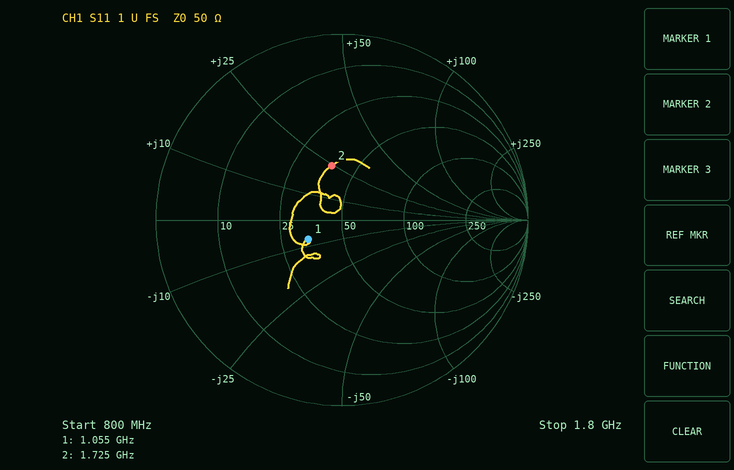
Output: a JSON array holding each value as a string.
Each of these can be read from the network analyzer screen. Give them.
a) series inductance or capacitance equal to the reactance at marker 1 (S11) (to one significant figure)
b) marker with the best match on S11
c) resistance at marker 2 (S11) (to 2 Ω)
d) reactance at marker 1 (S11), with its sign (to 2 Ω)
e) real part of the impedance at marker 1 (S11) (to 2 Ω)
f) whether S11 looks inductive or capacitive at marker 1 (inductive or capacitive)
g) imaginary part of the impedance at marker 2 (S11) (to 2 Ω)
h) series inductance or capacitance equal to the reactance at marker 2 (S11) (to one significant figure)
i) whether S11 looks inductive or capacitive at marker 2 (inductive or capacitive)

["20 pF", "marker 1", "38 Ω", "-8 Ω", "34 Ω", "capacitive", "+24 Ω", "2 nH", "inductive"]
